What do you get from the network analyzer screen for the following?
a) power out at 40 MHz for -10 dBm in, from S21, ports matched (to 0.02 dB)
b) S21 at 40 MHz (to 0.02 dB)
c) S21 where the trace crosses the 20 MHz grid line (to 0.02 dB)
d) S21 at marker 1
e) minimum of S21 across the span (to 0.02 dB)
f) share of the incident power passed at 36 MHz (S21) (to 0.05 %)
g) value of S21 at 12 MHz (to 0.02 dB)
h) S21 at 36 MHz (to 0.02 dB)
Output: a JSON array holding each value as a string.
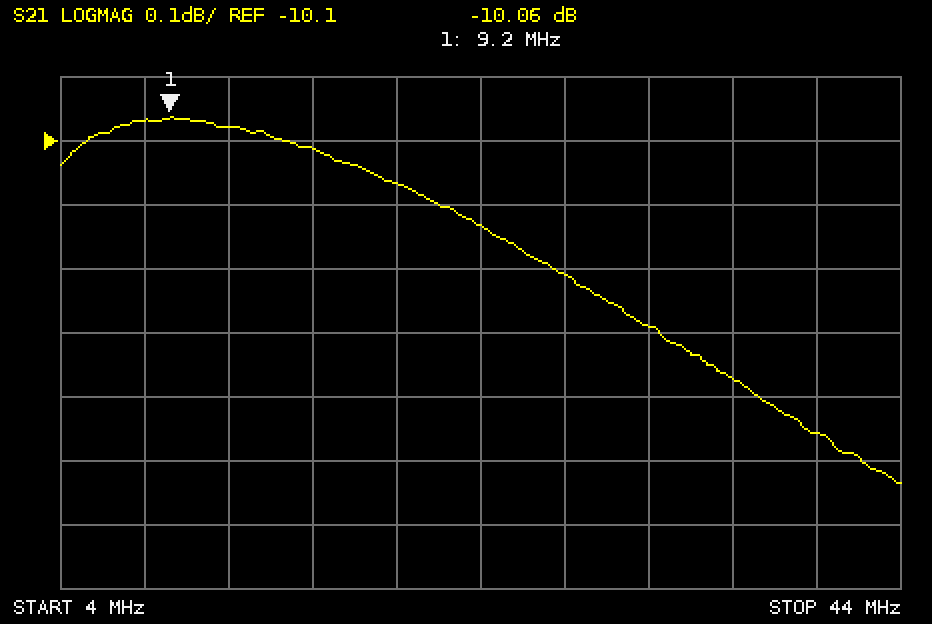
["-20.56 dBm", "-10.56 dB", "-10.16 dB", "-10.06 dB", "-10.64 dB", "8.95 %", "-10.08 dB", "-10.48 dB"]
